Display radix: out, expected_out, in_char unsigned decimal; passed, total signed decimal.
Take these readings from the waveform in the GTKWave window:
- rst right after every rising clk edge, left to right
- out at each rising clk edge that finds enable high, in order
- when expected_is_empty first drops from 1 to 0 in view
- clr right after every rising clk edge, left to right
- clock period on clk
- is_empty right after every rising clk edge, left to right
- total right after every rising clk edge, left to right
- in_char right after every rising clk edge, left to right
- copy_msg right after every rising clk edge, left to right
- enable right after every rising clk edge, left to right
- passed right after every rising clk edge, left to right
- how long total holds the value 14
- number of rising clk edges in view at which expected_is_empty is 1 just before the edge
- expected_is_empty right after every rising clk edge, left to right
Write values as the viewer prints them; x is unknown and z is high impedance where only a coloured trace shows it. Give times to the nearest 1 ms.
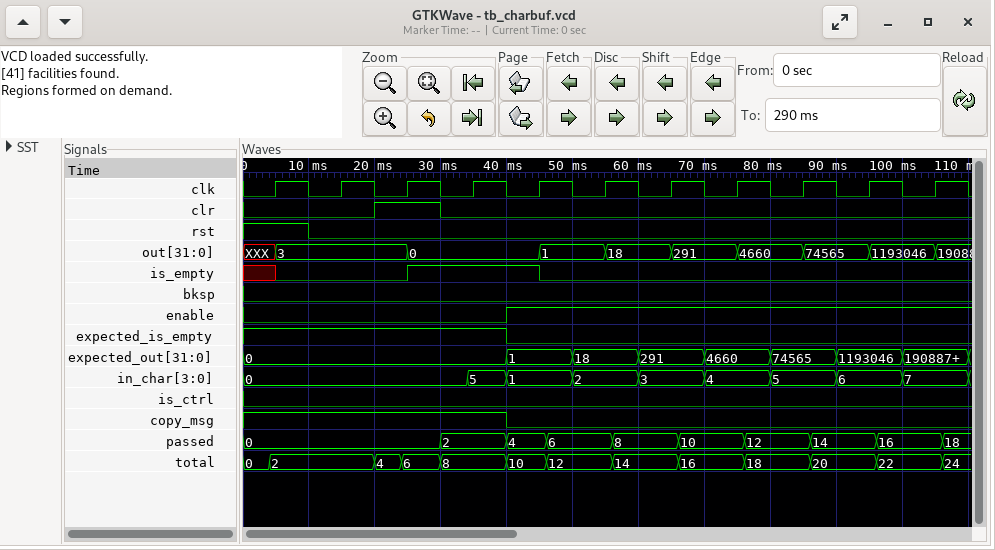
1 0 0 0 0 0 0 0 0 0 0
0, 1, 18, 291, 4660, 74565, 1193046
40 ms
0 0 1 0 0 0 0 0 0 0 0
10 ms
0 0 1 1 0 0 0 0 0 0 0
2, 2, 6, 8, 10, 12, 14, 16, 18, 20, 22
0, 0, 0, 5, 1, 2, 3, 4, 5, 6, 7
1 1 1 1 0 0 0 0 0 0 0
0 0 0 0 1 1 1 1 1 1 1
0, 0, 0, 2, 4, 6, 8, 10, 12, 14, 16
10 ms
4
1 1 1 1 0 0 0 0 0 0 0
